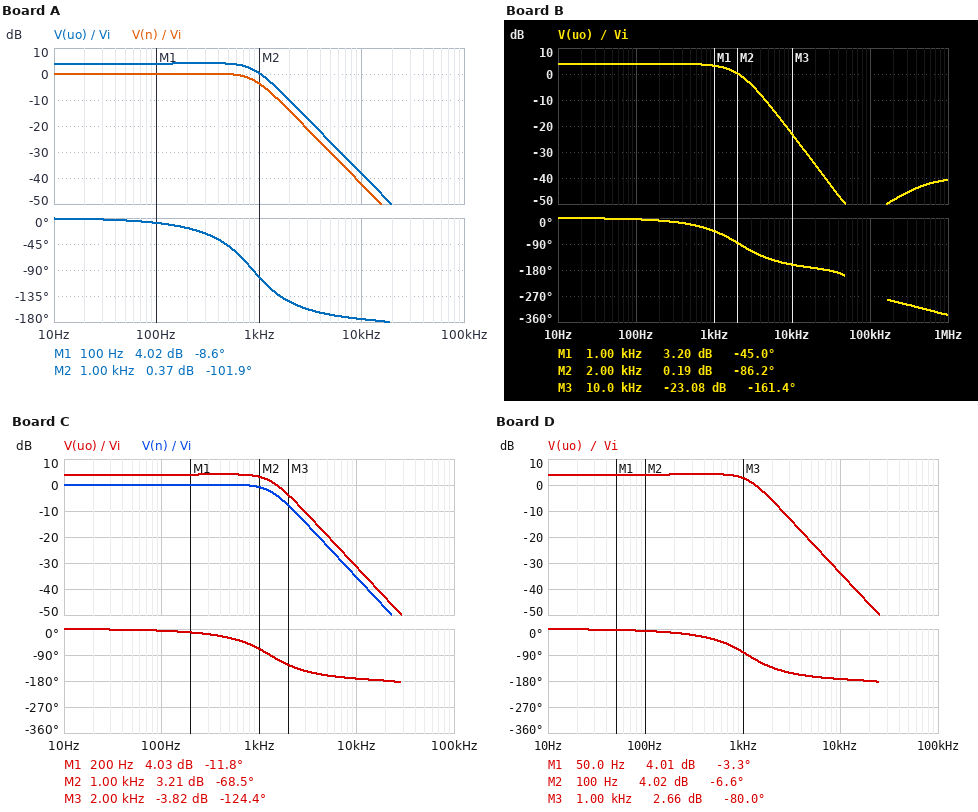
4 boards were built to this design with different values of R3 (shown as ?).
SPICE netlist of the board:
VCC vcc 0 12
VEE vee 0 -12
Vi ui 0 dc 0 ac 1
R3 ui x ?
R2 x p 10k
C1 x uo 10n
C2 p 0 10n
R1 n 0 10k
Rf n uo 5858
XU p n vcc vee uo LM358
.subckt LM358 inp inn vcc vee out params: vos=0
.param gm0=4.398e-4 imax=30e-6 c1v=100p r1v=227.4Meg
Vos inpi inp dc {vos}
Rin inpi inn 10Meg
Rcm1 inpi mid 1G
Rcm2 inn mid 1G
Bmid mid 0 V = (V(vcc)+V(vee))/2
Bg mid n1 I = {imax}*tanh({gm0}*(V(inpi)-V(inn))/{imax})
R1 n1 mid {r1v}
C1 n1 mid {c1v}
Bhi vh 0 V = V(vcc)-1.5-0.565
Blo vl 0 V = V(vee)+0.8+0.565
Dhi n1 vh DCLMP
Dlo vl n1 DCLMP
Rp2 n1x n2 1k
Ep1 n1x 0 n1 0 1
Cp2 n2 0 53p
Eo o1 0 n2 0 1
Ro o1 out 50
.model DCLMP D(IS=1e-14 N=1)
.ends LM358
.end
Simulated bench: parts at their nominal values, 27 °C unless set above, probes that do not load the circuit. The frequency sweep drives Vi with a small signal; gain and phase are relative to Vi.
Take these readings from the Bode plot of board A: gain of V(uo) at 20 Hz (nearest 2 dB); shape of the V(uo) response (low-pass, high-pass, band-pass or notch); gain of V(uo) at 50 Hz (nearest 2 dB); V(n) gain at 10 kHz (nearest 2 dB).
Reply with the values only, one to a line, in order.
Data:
4 dB
low-pass
4 dB
-42 dB
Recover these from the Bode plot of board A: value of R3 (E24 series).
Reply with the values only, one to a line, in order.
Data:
33 kΩ
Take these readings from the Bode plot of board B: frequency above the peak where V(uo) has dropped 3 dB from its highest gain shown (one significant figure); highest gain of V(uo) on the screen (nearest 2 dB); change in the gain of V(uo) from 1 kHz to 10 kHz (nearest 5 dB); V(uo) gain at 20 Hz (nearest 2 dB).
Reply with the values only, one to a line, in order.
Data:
2 kHz
4 dB
-25 dB
4 dB
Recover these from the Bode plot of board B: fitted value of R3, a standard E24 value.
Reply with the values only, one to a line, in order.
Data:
5.6 kΩ
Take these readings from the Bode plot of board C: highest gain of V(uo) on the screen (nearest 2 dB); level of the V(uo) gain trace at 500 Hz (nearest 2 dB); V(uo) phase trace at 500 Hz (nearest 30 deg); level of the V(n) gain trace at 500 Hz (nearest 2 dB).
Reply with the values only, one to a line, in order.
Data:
4 dB
4 dB
-30 deg
0 dB
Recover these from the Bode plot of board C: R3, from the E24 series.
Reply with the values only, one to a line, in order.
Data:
15 kΩ
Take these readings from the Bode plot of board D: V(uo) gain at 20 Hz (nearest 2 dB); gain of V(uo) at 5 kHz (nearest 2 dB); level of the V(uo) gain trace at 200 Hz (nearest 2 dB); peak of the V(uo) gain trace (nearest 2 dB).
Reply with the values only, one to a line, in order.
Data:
4 dB
-22 dB
4 dB
4 dB
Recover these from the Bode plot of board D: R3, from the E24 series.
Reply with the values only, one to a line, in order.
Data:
20 kΩ
